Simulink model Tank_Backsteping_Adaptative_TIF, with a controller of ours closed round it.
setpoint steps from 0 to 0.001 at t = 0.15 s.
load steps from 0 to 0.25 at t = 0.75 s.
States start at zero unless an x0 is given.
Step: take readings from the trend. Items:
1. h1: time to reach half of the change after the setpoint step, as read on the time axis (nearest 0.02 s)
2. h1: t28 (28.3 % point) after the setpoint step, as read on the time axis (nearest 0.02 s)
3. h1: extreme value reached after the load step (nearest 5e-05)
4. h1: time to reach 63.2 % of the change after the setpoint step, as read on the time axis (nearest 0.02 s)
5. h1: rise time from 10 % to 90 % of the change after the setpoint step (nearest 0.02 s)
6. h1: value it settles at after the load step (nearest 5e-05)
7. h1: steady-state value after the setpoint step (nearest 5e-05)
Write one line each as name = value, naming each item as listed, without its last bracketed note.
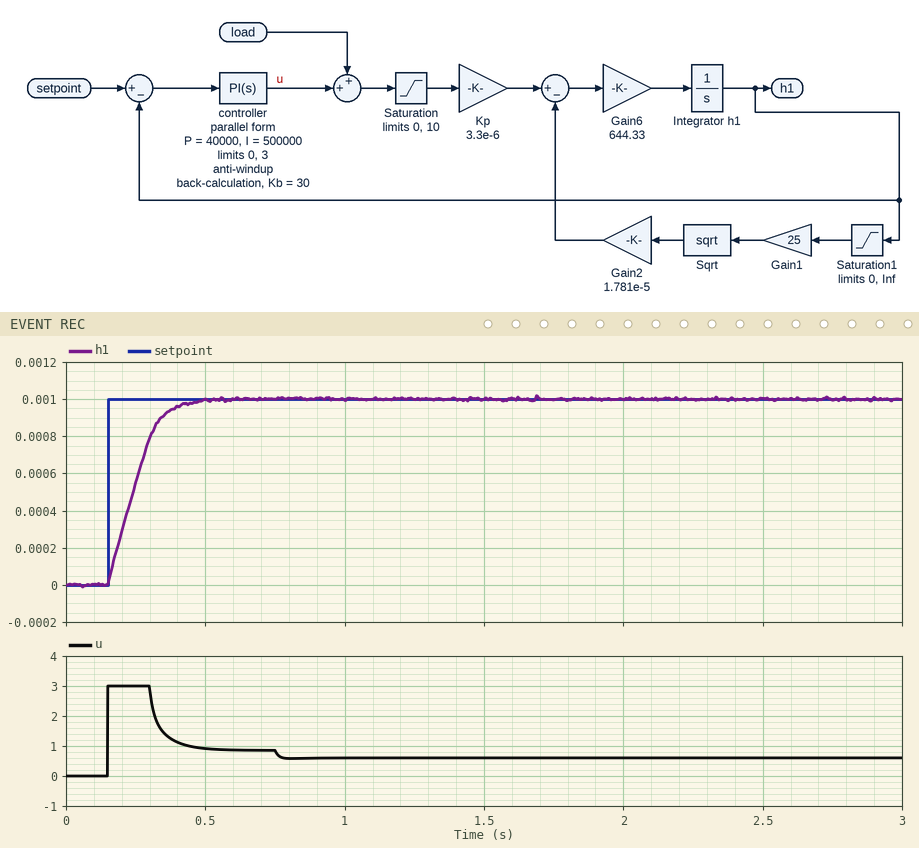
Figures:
h1: time to reach half of the change after the setpoint step, as read on the time axis = 0.24 s
h1: t28 (28.3 % point) after the setpoint step, as read on the time axis = 0.20 s
h1: extreme value reached after the load step = 0.00100
h1: time to reach 63.2 % of the change after the setpoint step, as read on the time axis = 0.26 s
h1: rise time from 10 % to 90 % of the change after the setpoint step = 0.18 s
h1: value it settles at after the load step = 0.00100
h1: steady-state value after the setpoint step = 0.00100
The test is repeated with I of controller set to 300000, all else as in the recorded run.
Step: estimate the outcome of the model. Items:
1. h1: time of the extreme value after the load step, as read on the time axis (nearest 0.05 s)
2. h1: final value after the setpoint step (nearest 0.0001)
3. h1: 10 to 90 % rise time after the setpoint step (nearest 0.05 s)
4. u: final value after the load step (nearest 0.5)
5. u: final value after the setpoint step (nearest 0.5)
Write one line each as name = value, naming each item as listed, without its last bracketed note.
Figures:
h1: time of the extreme value after the load step, as read on the time axis = 0.80 s
h1: final value after the setpoint step = 0.0010
h1: 10 to 90 % rise time after the setpoint step = 0.25 s
u: final value after the load step = 0.5
u: final value after the setpoint step = 1.0
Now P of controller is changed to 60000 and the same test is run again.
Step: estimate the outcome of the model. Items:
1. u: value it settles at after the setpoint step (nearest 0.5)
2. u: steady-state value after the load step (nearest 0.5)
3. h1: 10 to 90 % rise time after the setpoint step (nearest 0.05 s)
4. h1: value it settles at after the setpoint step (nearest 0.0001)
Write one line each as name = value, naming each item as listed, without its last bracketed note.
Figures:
u: value it settles at after the setpoint step = 1.0
u: steady-state value after the load step = 0.5
h1: 10 to 90 % rise time after the setpoint step = 0.25 s
h1: value it settles at after the setpoint step = 0.0010
